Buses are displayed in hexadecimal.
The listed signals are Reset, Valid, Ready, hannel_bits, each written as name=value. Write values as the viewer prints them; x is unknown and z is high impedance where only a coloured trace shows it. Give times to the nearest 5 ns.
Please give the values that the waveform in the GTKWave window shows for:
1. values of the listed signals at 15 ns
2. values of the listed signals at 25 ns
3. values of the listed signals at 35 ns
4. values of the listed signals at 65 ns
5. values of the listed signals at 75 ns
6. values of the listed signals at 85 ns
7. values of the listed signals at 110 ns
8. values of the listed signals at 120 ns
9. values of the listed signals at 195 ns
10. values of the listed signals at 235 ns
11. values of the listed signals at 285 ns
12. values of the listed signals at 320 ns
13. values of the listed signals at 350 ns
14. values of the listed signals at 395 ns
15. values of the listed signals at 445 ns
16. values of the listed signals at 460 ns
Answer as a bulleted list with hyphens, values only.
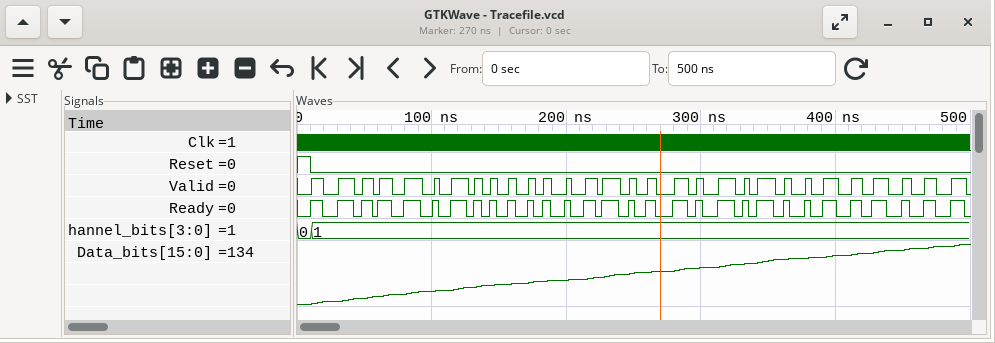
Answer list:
- Reset=0, Valid=1, Ready=1, hannel_bits=1
- Reset=0, Valid=0, Ready=0, hannel_bits=1
- Reset=0, Valid=1, Ready=1, hannel_bits=1
- Reset=0, Valid=1, Ready=1, hannel_bits=1
- Reset=0, Valid=0, Ready=0, hannel_bits=1
- Reset=0, Valid=1, Ready=1, hannel_bits=1
- Reset=0, Valid=0, Ready=0, hannel_bits=1
- Reset=0, Valid=1, Ready=1, hannel_bits=1
- Reset=0, Valid=0, Ready=0, hannel_bits=1
- Reset=0, Valid=1, Ready=1, hannel_bits=1
- Reset=0, Valid=1, Ready=1, hannel_bits=1
- Reset=0, Valid=1, Ready=1, hannel_bits=1
- Reset=0, Valid=1, Ready=1, hannel_bits=1
- Reset=0, Valid=1, Ready=1, hannel_bits=1
- Reset=0, Valid=0, Ready=0, hannel_bits=1
- Reset=0, Valid=0, Ready=0, hannel_bits=1
